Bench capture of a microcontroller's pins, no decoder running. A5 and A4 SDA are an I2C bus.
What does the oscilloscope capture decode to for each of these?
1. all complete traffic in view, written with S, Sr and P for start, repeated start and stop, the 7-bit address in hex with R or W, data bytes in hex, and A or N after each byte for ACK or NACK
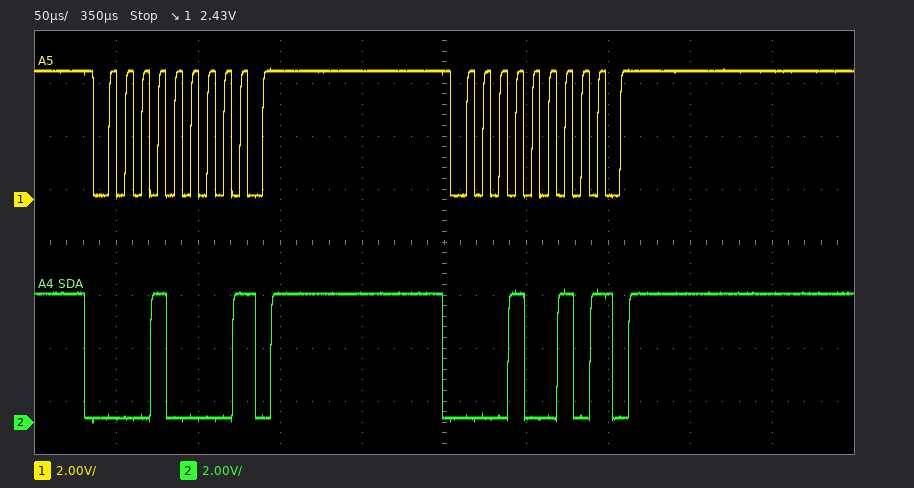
S 08W N P S 09W N P
